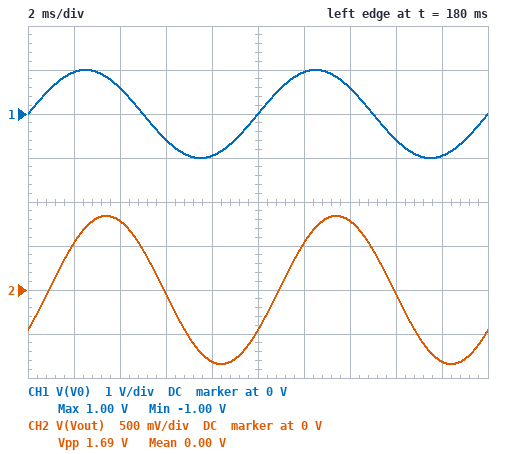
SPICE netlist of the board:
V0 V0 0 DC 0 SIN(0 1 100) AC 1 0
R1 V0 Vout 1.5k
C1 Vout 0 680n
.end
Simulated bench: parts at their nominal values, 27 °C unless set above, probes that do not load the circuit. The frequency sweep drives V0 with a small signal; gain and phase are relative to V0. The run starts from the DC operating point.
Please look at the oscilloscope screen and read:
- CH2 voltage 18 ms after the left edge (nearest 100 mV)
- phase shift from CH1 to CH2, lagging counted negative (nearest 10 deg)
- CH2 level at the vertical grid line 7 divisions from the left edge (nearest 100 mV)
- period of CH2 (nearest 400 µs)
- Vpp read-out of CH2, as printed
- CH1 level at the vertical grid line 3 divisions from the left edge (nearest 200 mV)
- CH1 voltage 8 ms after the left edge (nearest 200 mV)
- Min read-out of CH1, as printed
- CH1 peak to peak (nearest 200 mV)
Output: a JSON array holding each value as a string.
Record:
["-800 mV", "-30 deg", "800 mV", "10.0 ms", "1.69 V", "-600 mV", "-1.0 V", "-1.00 V", "2.0 V"]
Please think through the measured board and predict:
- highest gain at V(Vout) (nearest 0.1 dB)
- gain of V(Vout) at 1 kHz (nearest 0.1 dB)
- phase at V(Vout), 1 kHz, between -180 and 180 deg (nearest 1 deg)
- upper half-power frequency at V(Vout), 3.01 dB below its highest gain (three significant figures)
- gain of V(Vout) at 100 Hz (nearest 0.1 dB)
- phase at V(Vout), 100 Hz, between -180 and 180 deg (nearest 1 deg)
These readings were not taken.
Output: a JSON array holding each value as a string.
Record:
["0 dB", "-16.2 dB", "-81 deg", "156 Hz", "-1.5 dB", "-33 deg"]
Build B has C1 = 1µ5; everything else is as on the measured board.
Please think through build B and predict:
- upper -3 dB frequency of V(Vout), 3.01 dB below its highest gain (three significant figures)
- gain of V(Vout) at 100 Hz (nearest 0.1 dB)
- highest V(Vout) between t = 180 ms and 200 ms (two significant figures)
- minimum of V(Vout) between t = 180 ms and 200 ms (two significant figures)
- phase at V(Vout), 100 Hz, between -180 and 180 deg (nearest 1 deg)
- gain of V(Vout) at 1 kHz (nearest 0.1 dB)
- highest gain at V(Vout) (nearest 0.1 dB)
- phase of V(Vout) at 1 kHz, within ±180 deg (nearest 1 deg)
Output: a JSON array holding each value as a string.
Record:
["70.7 Hz", "-4.8 dB", "580 mV", "-580 mV", "-55 deg", "-23.0 dB", "0 dB", "-86 deg"]
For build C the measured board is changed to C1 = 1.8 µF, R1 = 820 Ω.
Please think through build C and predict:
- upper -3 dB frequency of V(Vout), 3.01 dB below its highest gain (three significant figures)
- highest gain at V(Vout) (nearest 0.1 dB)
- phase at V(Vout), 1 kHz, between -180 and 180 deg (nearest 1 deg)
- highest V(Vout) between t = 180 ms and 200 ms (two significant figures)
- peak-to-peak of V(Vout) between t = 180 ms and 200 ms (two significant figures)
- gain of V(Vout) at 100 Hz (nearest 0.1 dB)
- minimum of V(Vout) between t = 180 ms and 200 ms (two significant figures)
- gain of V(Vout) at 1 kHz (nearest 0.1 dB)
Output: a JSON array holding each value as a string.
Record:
["108 Hz", "0 dB", "-84 deg", "730 mV", "1.5 V", "-2.7 dB", "-730 mV", "-19.4 dB"]
